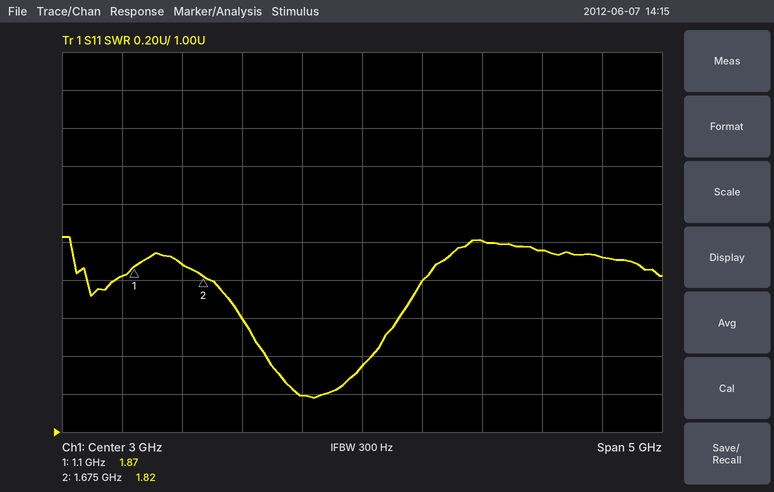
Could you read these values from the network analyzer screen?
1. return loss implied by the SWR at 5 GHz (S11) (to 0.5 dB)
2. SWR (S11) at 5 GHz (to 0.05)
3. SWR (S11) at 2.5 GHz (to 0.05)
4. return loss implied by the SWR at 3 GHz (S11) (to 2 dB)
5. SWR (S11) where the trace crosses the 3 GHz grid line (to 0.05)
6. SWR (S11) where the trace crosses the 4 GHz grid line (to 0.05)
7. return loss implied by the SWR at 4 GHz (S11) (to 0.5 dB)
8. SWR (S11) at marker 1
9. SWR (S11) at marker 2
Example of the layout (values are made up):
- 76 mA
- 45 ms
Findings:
- 10.0 dB
- 1.90
- 1.20
- 16 dB
- 1.35
- 2.00
- 9.5 dB
- 1.87
- 1.82
